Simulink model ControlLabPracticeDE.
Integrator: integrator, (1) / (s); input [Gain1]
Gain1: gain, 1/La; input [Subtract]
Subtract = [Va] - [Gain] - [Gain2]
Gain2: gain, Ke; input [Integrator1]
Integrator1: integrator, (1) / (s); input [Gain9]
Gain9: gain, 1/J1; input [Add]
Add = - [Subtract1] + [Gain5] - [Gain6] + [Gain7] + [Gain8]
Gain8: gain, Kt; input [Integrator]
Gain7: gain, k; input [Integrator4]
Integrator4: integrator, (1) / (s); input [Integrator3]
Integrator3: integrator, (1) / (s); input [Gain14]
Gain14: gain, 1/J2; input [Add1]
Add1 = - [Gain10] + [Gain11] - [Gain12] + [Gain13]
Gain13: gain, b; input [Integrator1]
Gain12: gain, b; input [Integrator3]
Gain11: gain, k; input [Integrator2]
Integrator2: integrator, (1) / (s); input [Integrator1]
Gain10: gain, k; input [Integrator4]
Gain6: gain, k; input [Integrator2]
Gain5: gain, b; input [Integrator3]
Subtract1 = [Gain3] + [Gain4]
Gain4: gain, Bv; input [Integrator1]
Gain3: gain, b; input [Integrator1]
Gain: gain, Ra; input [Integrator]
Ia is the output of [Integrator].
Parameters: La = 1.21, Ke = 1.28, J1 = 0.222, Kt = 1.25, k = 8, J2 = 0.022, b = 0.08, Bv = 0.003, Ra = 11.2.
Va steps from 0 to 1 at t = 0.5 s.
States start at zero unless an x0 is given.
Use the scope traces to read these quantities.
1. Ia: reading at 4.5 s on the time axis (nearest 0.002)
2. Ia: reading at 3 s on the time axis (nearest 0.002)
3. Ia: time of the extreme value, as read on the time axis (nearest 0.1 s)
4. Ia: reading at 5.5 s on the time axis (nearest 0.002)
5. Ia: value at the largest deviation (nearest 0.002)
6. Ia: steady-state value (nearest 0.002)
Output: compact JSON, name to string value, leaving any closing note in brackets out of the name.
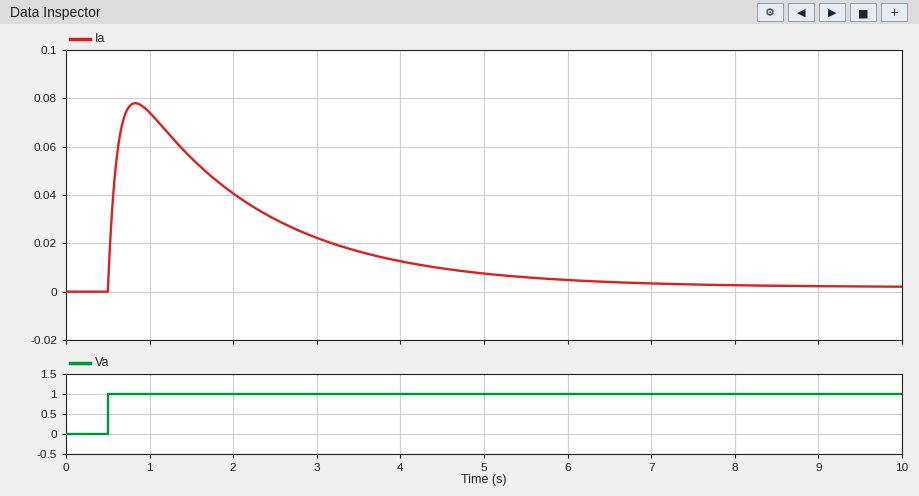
{"Ia: reading at 4.5 s on the time axis": "0.010", "Ia: reading at 3 s on the time axis": "0.022", "Ia: time of the extreme value, as read on the time axis": "0.8 s", "Ia: reading at 5.5 s on the time axis": "0.006", "Ia: value at the largest deviation": "0.078", "Ia: steady-state value": "0.002"}
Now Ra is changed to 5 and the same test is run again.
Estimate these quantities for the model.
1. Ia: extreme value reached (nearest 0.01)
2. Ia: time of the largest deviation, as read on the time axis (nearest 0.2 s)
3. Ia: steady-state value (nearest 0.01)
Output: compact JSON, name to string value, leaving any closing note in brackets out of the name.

{"Ia: extreme value reached": "0.14", "Ia: time of the largest deviation, as read on the time axis": "1.0 s", "Ia: steady-state value": "0.00"}
